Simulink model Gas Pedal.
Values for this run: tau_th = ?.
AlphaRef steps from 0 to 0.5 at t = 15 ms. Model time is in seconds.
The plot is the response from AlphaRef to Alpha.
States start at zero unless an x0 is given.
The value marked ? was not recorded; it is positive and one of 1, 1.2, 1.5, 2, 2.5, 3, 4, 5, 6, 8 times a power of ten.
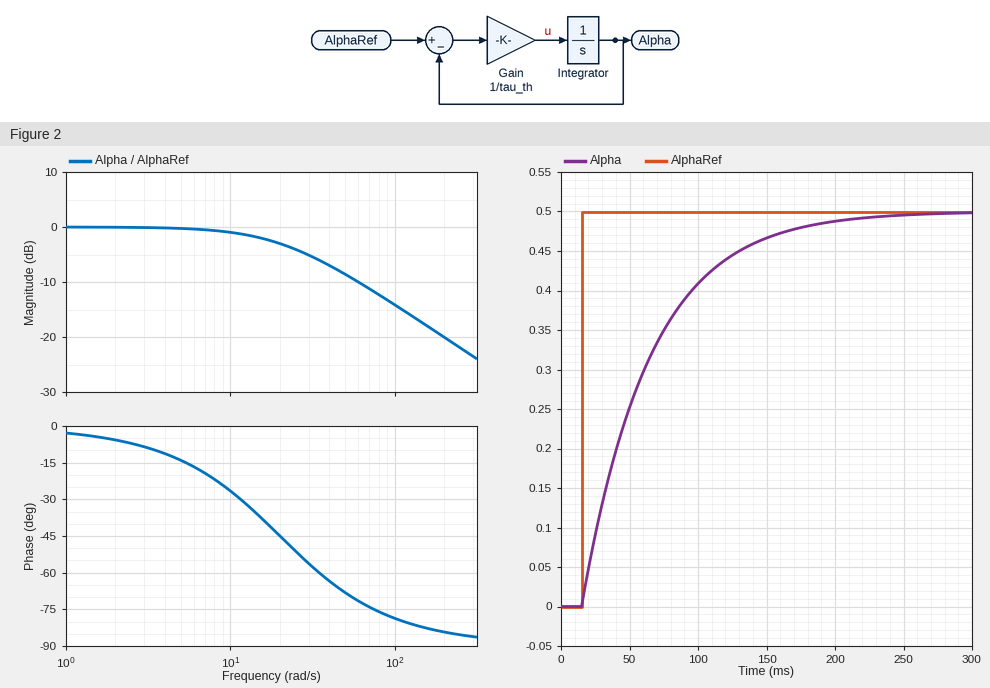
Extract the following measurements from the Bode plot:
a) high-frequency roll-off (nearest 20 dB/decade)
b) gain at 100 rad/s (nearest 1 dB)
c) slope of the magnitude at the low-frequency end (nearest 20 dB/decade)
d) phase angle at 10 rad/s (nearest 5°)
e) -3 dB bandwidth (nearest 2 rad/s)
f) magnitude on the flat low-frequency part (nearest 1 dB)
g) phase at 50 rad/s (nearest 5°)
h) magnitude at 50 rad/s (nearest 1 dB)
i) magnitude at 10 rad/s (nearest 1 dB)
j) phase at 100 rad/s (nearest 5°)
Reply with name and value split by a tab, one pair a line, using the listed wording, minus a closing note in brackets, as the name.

high-frequency roll-off	-20 dB/decade
gain at 100 rad/s	-14 dB
slope of the magnitude at the low-frequency end	0 dB/decade
phase angle at 10 rad/s	-25°
-3 dB bandwidth	20 rad/s
magnitude on the flat low-frequency part	0 dB
phase at 50 rad/s	-70°
magnitude at 50 rad/s	-9 dB
magnitude at 10 rad/s	-1 dB
phase at 100 rad/s	-80°
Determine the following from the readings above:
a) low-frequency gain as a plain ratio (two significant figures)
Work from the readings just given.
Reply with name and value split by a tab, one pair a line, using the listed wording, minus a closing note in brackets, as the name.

low-frequency gain as a plain ratio	1.0
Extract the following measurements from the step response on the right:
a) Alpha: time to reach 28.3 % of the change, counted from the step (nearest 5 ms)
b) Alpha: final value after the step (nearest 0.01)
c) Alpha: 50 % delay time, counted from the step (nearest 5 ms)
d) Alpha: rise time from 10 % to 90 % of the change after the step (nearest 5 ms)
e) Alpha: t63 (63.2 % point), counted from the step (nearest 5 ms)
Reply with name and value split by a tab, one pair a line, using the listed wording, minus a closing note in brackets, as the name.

Alpha: time to reach 28.3 % of the change, counted from the step	15 ms
Alpha: final value after the step	0.50
Alpha: 50 % delay time, counted from the step	35 ms
Alpha: rise time from 10 % to 90 % of the change after the step	110 ms
Alpha: t63 (63.2 % point), counted from the step	50 ms
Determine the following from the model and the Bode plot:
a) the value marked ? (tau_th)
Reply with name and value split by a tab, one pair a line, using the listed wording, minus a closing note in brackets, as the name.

the value marked ?	0.05
